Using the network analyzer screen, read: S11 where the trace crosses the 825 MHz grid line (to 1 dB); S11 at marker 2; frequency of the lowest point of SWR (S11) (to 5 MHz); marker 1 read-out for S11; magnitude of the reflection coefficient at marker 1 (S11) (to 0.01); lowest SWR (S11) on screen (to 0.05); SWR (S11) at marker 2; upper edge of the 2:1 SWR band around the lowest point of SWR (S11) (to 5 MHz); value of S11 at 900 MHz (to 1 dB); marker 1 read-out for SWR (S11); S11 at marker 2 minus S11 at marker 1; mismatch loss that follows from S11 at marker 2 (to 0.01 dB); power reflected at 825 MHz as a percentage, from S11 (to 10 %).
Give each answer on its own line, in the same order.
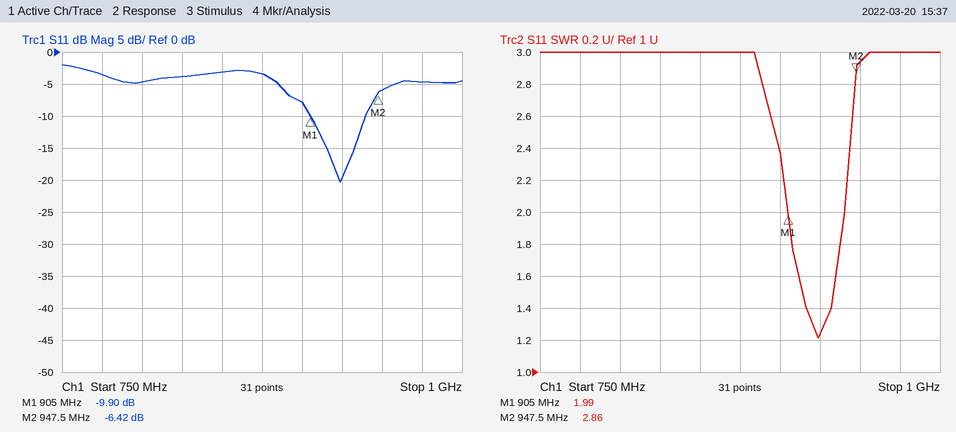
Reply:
-4 dB
-6.42 dB
925 MHz
-9.90 dB
0.32
1.20
2.86
940 MHz
-8 dB
1.99
3.48 dB
1.12 dB
40 %
